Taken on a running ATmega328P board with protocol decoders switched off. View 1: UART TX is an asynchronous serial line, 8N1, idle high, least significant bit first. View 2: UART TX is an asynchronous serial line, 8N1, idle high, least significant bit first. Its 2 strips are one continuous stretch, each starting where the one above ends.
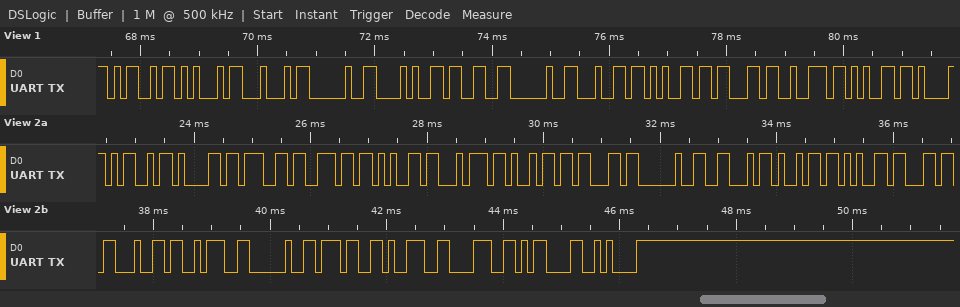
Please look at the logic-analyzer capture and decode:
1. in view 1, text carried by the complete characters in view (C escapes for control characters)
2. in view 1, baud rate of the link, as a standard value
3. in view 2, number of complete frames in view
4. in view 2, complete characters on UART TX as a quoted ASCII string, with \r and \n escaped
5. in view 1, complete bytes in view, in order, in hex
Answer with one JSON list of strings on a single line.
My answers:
["\"MED (3 decre\"", "9600 baud", "21", "\"Magnetic Field: 798\\r\\n\"", "0x4D 0x45 0x44 0x20 0x28 0x33 0x20 0x64 0x65 0x63 0x72 0x65"]
